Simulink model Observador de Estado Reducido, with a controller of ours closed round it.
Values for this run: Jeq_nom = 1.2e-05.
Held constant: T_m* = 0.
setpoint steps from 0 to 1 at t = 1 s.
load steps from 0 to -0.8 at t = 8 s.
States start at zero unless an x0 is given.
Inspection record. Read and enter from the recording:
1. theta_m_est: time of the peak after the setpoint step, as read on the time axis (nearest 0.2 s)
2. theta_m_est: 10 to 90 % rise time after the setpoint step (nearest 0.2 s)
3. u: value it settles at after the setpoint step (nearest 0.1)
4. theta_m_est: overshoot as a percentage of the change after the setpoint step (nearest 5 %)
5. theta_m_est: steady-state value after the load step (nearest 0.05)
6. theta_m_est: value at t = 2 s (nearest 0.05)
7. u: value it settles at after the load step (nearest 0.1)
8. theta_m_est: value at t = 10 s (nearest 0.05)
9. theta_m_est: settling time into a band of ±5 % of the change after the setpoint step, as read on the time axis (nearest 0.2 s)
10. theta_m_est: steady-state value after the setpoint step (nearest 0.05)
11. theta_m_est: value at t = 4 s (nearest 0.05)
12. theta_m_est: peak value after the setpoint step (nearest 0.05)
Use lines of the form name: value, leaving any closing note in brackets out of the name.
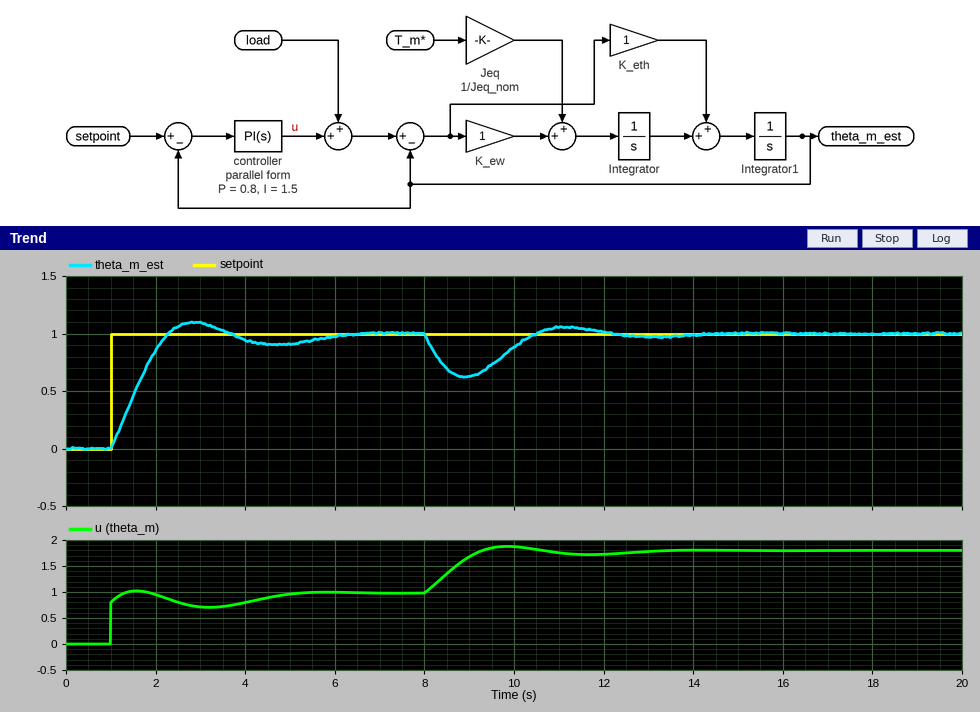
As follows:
theta_m_est: time of the peak after the setpoint step, as read on the time axis: 2.8 s
theta_m_est: 10 to 90 % rise time after the setpoint step: 1.0 s
u: value it settles at after the setpoint step: 1.0
theta_m_est: overshoot as a percentage of the change after the setpoint step: 10 %
theta_m_est: steady-state value after the load step: 1.00
theta_m_est: value at t = 2 s: 0.85
u: value it settles at after the load step: 1.8
theta_m_est: value at t = 10 s: 0.90
theta_m_est: settling time into a band of ±5 % of the change after the setpoint step, as read on the time axis: 5.6 s
theta_m_est: steady-state value after the setpoint step: 1.00
theta_m_est: value at t = 4 s: 0.95
theta_m_est: peak value after the setpoint step: 1.10
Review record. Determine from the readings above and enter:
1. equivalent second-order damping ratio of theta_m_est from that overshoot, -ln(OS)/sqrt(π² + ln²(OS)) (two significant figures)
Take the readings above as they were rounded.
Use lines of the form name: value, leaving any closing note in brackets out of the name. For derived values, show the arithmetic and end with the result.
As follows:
equivalent second-order damping ratio of theta_m_est from that overshoot, -ln(OS)/sqrt(π² + ln²(OS)): ln(0.1) = -2.303; 2.303 / sqrt(9.870 + 5.302) = 0.59
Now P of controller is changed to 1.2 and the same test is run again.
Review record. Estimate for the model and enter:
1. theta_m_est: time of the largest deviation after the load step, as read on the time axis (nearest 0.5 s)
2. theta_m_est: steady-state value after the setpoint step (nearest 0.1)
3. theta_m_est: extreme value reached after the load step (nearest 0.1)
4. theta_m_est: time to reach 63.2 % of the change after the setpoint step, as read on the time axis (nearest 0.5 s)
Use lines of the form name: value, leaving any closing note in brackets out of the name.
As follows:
theta_m_est: time of the largest deviation after the load step, as read on the time axis: 9.0 s
theta_m_est: steady-state value after the setpoint step: 1.0
theta_m_est: extreme value reached after the load step: 0.7
theta_m_est: time to reach 63.2 % of the change after the setpoint step, as read on the time axis: 1.5 s
